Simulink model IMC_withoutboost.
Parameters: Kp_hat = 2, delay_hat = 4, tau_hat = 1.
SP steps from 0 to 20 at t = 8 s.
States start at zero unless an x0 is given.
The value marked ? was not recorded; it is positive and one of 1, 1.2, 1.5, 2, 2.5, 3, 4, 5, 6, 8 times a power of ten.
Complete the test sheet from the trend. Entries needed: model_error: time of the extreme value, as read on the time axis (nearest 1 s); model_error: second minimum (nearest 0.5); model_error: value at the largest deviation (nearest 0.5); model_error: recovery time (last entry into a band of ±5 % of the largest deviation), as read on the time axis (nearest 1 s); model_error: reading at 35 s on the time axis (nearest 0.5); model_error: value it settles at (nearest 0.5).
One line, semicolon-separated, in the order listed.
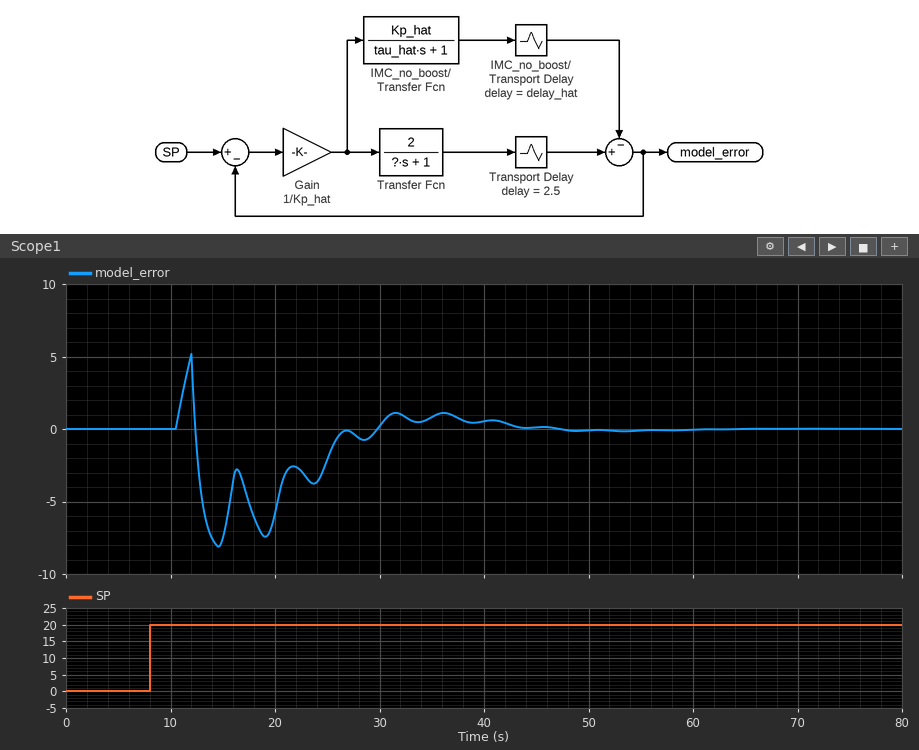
15 s; -7.5; -8.0; 42 s; 1.0; 0.0
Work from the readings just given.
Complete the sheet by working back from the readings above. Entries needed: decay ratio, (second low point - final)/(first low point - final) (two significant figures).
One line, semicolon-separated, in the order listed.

0.94
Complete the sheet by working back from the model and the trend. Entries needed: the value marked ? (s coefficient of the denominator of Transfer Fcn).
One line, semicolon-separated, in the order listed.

5
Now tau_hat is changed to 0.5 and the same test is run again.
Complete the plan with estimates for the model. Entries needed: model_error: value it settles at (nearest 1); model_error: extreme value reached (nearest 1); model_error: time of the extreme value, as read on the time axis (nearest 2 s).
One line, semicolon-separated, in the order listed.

0; -10; 18 s
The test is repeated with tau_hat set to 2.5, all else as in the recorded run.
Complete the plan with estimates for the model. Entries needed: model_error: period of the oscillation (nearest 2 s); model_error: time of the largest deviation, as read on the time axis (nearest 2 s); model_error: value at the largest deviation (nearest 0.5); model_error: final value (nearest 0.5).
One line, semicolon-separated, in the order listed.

6 s; 12 s; 5.0; 0.0
